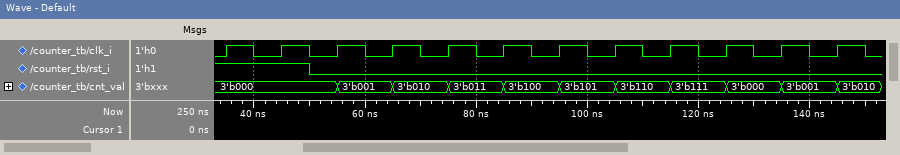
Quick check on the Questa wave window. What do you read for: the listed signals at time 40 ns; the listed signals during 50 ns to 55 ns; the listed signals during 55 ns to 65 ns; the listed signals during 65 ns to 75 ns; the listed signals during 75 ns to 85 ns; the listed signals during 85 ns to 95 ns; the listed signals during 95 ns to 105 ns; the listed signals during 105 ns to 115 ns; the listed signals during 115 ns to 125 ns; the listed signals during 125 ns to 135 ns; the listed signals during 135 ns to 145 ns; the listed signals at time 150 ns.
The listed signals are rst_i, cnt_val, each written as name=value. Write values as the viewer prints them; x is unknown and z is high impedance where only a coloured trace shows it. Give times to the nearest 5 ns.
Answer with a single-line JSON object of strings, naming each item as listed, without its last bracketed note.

{"the listed signals at time 40 ns": "rst_i=1, cnt_val=3'b000", "the listed signals during 50 ns to 55 ns": "rst_i=0, cnt_val=3'b000", "the listed signals during 55 ns to 65 ns": "rst_i=0, cnt_val=3'b001", "the listed signals during 65 ns to 75 ns": "rst_i=0, cnt_val=3'b010", "the listed signals during 75 ns to 85 ns": "rst_i=0, cnt_val=3'b011", "the listed signals during 85 ns to 95 ns": "rst_i=0, cnt_val=3'b100", "the listed signals during 95 ns to 105 ns": "rst_i=0, cnt_val=3'b101", "the listed signals during 105 ns to 115 ns": "rst_i=0, cnt_val=3'b110", "the listed signals during 115 ns to 125 ns": "rst_i=0, cnt_val=3'b111", "the listed signals during 125 ns to 135 ns": "rst_i=0, cnt_val=3'b000", "the listed signals during 135 ns to 145 ns": "rst_i=0, cnt_val=3'b001", "the listed signals at time 150 ns": "rst_i=0, cnt_val=3'b010"}
